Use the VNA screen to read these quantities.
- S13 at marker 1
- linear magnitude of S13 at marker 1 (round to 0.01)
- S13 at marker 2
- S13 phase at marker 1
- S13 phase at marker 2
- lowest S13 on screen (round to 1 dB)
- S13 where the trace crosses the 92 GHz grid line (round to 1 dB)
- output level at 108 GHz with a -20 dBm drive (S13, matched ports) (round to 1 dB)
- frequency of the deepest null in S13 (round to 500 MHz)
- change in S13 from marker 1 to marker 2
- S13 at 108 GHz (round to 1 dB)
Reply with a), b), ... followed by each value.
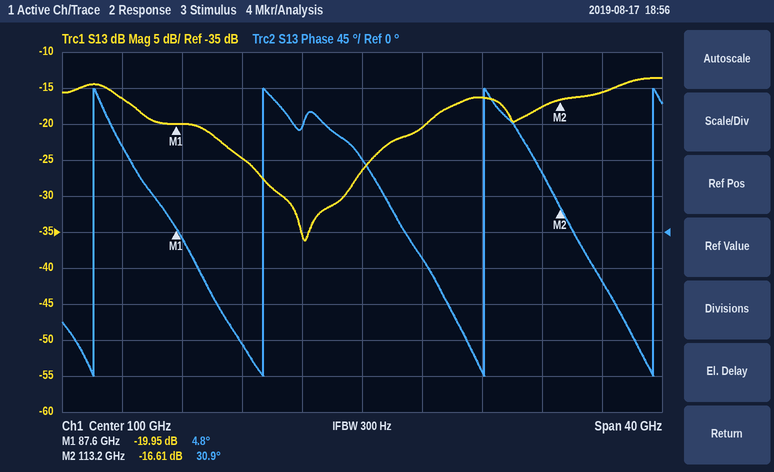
a) -19.95 dB
b) 0.10
c) -16.61 dB
d) 4.8°
e) 30.9°
f) -36 dB
g) -25 dB
h) -36 dBm
i) 96.0 GHz
j) 3.34 dB
k) -16 dB
